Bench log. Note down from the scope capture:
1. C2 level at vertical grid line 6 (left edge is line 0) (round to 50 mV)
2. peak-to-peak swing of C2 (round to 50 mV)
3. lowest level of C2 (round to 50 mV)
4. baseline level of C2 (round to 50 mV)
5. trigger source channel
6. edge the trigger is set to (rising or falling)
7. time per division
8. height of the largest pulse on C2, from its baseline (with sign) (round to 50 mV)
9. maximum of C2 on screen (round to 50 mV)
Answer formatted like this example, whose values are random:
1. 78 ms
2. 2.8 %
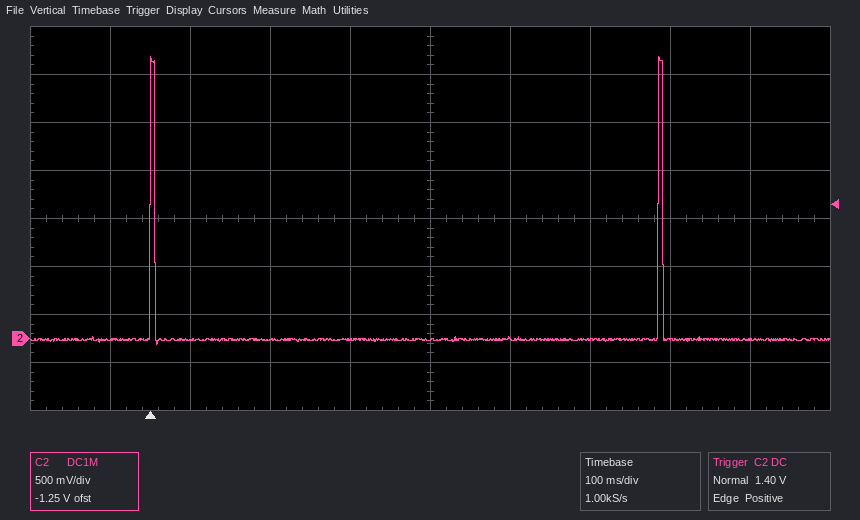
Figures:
1. 0 mV
2. 3.00 V
3. -50 mV
4. 0 mV
5. C2
6. rising
7. 100 ms
8. +2.95 V
9. 2.95 V
